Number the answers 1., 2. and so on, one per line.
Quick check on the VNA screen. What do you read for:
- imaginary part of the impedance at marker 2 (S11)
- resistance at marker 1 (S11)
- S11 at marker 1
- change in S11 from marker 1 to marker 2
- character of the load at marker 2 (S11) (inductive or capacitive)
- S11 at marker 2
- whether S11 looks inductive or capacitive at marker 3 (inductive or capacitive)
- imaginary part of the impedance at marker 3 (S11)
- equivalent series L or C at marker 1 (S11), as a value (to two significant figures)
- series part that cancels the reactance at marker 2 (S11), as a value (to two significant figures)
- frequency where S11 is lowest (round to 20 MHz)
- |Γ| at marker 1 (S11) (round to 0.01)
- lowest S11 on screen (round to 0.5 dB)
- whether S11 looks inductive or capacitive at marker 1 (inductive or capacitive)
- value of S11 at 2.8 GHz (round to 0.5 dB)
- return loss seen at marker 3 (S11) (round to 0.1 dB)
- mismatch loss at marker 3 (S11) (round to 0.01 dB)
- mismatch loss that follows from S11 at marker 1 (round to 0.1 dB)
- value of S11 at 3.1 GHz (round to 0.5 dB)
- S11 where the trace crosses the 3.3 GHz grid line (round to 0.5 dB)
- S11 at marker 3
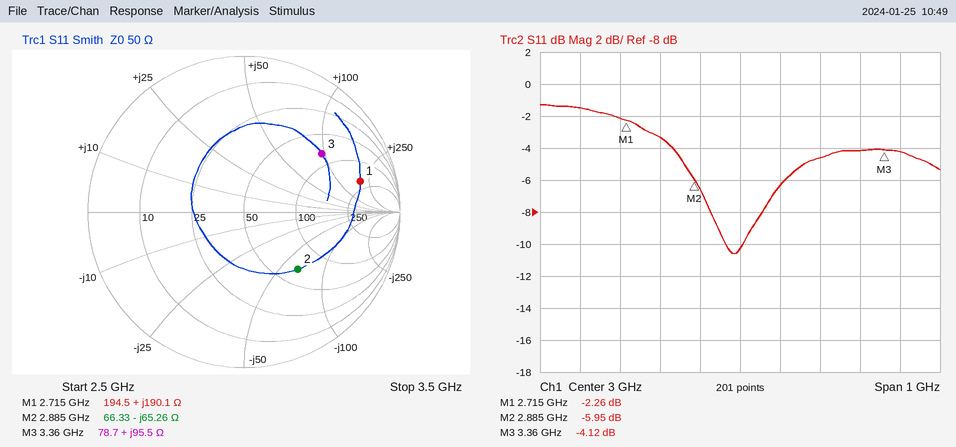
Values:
1. -65.26 Ω
2. 194.5 Ω
3. -2.26 dB
4. -3.69 dB
5. capacitive
6. -5.95 dB
7. inductive
8. +95.5 Ω
9. 11 nH
10. 3.6 nH
11. 2.98 GHz
12. 0.77
13. -10.5 dB
14. inductive
15. -3.5 dB
16. 4.1 dB
17. 2.13 dB
18. 3.9 dB
19. -6.5 dB
20. -4.0 dB
21. -4.12 dB
